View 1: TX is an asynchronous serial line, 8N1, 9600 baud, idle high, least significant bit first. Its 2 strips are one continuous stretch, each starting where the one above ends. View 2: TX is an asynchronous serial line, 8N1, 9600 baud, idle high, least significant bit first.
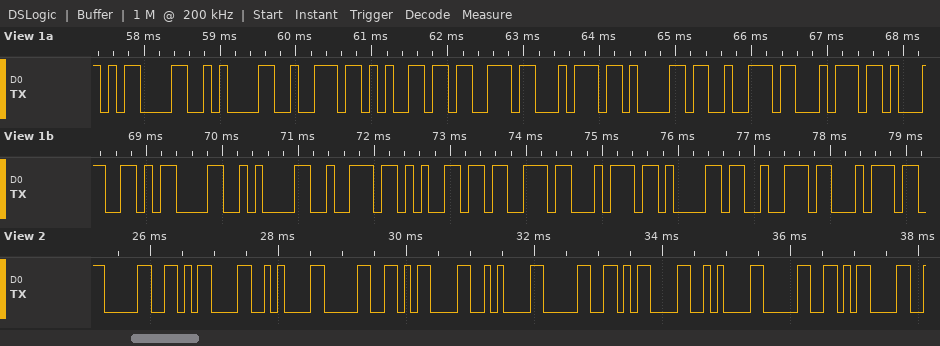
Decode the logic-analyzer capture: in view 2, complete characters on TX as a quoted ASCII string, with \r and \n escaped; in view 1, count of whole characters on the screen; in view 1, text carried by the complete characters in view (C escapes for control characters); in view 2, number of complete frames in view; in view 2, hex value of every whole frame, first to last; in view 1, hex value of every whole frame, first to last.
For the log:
"0\r\n0\r\n0\r\n0\r"
19
"\r\nrestart1\r\nrestart"
11
0x30 0x0D 0x0A 0x30 0x0D 0x0A 0x30 0x0D 0x0A 0x30 0x0D
0D 0A 72 65 73 74 61 72 74 31 0D 0A 72 65 73 74 61 72 74
